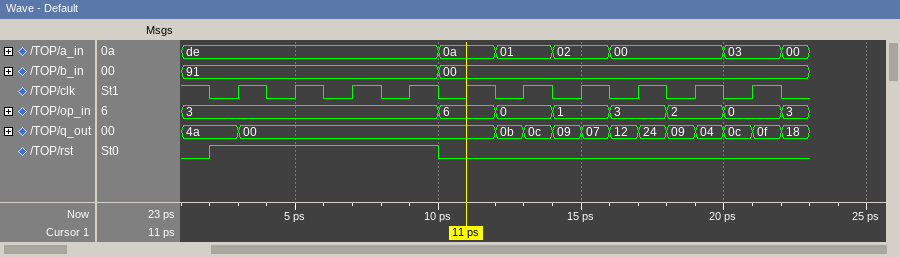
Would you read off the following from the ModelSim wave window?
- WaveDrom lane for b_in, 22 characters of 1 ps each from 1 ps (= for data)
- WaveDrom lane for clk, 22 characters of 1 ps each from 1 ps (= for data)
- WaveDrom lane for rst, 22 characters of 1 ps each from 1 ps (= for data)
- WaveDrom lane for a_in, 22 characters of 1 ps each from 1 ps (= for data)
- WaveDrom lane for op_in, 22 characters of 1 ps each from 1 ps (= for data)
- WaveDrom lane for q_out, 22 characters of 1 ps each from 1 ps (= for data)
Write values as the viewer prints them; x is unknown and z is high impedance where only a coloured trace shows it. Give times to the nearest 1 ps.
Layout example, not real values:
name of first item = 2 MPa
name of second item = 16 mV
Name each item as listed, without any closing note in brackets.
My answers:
WaveDrom lane for b_in, 22 characters of 1 ps each from 1 ps = {name: 'b_in', wave: '=........=............', data: '91 00'}
WaveDrom lane for clk, 22 characters of 1 ps each from 1 ps = {name: 'clk', wave: '1010101010101010101010'}
WaveDrom lane for rst, 22 characters of 1 ps each from 1 ps = {name: 'rst', wave: '01.......0............'}
WaveDrom lane for a_in, 22 characters of 1 ps each from 1 ps = {name: 'a_in', wave: '=........=.=.=.=...=.=', data: 'de 0a 01 02 00 03 00'}
WaveDrom lane for op_in, 22 characters of 1 ps each from 1 ps = {name: 'op_in', wave: '=........=.=.=.=.=.=.=', data: '3 6 0 1 3 2 0 3'}
WaveDrom lane for q_out, 22 characters of 1 ps each from 1 ps = {name: 'q_out', wave: '=.=........===========', data: '4a 00 0b 0c 09 07 12 24 09 04 0c 0f 18'}
